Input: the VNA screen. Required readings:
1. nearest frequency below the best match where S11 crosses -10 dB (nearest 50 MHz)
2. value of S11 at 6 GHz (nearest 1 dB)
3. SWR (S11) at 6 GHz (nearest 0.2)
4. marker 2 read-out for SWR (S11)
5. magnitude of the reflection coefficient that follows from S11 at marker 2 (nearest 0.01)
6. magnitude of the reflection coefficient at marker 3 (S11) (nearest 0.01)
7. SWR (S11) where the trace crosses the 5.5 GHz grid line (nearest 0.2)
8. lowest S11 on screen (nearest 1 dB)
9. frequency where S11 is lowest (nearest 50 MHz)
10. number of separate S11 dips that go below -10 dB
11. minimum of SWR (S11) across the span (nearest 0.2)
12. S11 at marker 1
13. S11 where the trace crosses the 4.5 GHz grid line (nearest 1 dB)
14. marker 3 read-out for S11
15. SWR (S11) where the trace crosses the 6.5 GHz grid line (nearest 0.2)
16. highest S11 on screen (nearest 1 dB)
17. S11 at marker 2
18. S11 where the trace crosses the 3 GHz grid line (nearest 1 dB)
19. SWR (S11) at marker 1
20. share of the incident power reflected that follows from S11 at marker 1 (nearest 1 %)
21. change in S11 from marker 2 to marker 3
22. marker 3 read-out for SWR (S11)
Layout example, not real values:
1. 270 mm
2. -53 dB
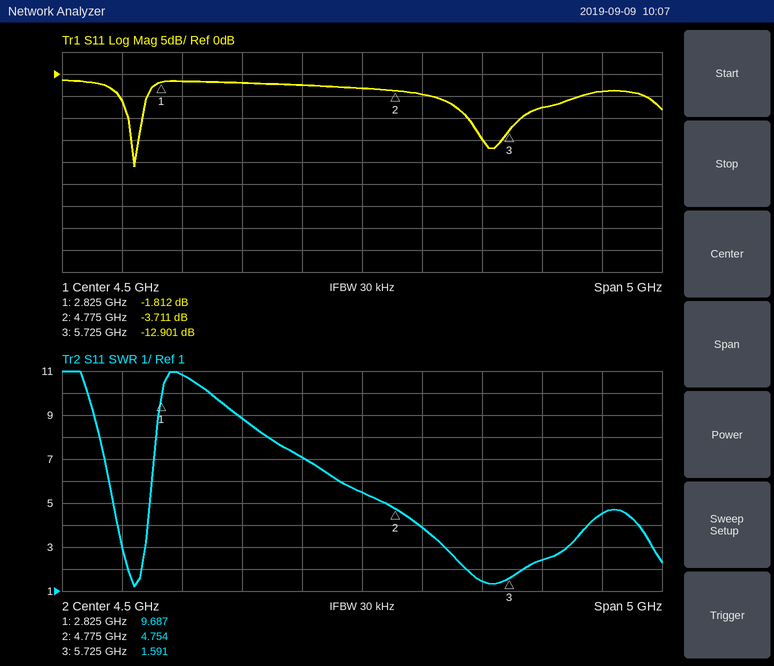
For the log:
1. 2.55 GHz
2. -8 dB
3. 2.4
4. 4.754
5. 0.65
6. 0.23
7. 1.4
8. -21 dB
9. 2.60 GHz
10. 2
11. 1.2
12. -1.812 dB
13. -3 dB
14. -12.901 dB
15. 4.6
16. -1 dB
17. -3.711 dB
18. -2 dB
19. 9.687
20. 66 %
21. -9.190 dB
22. 1.591
